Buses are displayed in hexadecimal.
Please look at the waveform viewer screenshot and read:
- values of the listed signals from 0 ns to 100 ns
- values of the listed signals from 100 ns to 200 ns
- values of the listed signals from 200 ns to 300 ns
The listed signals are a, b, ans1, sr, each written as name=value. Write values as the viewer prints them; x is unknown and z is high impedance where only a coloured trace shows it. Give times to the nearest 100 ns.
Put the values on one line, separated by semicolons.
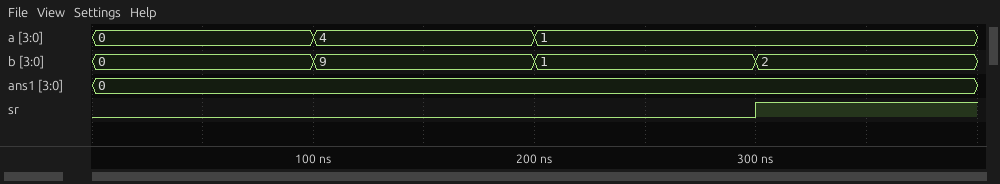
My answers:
a=0, b=0, ans1=0, sr=0; a=4, b=9, ans1=0, sr=0; a=1, b=1, ans1=0, sr=0
